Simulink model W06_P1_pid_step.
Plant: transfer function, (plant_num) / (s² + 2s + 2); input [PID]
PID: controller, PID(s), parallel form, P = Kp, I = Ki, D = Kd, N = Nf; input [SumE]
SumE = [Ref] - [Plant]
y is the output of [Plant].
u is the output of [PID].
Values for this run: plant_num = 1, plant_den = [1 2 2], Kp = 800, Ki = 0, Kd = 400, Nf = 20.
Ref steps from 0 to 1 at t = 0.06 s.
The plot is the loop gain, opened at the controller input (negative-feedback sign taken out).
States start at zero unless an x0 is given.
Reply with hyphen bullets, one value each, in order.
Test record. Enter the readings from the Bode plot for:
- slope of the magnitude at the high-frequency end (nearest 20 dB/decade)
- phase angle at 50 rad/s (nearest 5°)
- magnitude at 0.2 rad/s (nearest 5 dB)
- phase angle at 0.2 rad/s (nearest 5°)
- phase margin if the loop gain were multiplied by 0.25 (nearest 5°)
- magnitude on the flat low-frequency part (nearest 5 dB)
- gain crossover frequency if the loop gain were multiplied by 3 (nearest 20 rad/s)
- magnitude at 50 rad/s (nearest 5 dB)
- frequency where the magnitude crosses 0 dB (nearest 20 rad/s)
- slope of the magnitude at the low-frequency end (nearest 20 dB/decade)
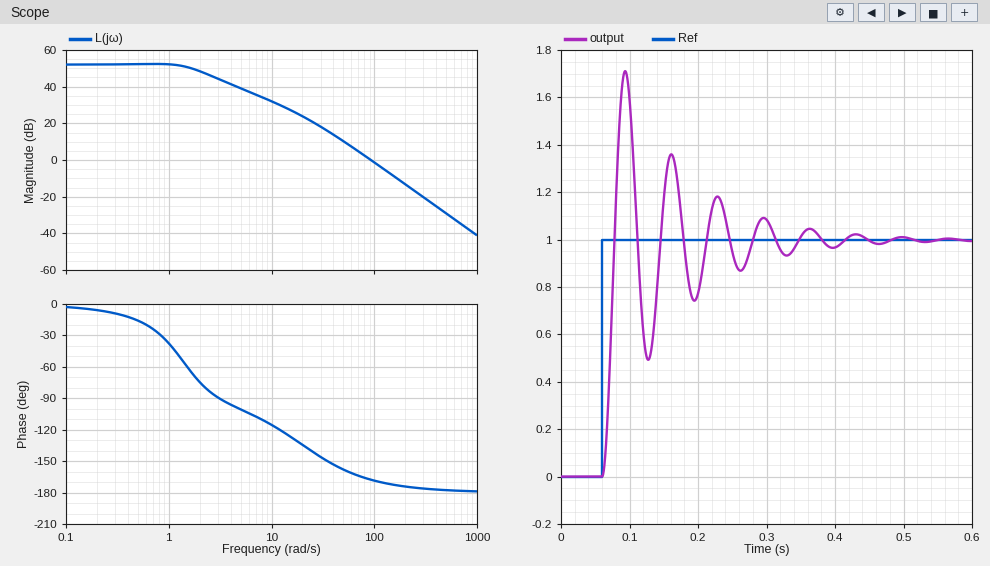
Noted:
- -40 dB/decade
- -160°
- 50 dB
- -5°
- 25°
- 50 dB
- 160 rad/s
- 10 dB
- 100 rad/s
- 0 dB/decade
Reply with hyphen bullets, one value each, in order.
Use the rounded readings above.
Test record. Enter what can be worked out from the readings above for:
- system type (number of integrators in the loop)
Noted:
- 0
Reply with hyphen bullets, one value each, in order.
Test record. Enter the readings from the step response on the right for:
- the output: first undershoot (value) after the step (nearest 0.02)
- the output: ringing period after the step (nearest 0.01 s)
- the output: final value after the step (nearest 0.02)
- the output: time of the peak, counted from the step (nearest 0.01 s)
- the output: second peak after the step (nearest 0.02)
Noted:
- 0.50
- 0.07 s
- 1.00
- 0.03 s
- 1.36
